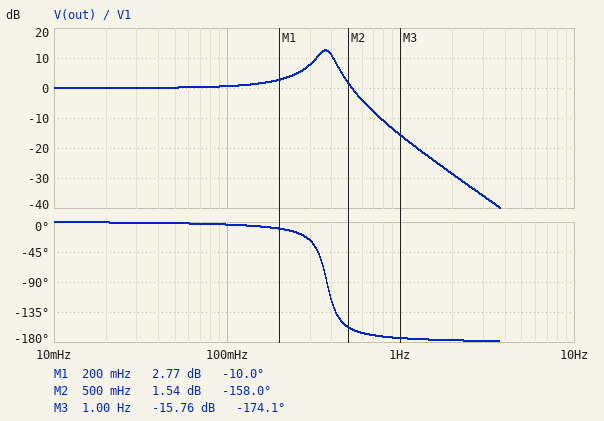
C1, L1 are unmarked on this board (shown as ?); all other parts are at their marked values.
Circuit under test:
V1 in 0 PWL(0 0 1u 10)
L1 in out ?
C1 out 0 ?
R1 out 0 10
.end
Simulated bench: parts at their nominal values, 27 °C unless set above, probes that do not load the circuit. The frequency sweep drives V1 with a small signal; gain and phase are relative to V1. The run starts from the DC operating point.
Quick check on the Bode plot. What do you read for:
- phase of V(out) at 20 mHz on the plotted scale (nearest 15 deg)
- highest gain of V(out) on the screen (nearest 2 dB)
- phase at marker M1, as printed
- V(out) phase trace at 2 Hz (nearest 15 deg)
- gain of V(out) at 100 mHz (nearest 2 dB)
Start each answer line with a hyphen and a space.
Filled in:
- 0 deg
- 12 dB
- -10.0 deg
- -180 deg
- 0 dB
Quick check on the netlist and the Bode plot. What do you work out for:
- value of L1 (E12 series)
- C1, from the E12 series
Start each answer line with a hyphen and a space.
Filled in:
- 1 H
- 180 mF
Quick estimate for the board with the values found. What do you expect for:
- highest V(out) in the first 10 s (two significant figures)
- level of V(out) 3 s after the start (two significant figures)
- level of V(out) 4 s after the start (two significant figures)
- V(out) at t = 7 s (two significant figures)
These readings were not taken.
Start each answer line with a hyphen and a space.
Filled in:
- 17 V
- 6.4 V
- 13 V
- 11 V
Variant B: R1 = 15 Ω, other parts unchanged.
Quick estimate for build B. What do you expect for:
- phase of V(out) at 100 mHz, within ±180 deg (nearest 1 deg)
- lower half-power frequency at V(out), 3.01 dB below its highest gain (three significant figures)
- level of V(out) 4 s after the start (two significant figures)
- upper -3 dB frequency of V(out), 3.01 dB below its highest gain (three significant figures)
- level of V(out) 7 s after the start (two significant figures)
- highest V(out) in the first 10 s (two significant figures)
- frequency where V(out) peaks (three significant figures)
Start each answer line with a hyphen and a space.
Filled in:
- -3 deg
- 342 mHz
- 15 V
- 401 mHz
- 12 V
- 18 V
- 373 mHz
